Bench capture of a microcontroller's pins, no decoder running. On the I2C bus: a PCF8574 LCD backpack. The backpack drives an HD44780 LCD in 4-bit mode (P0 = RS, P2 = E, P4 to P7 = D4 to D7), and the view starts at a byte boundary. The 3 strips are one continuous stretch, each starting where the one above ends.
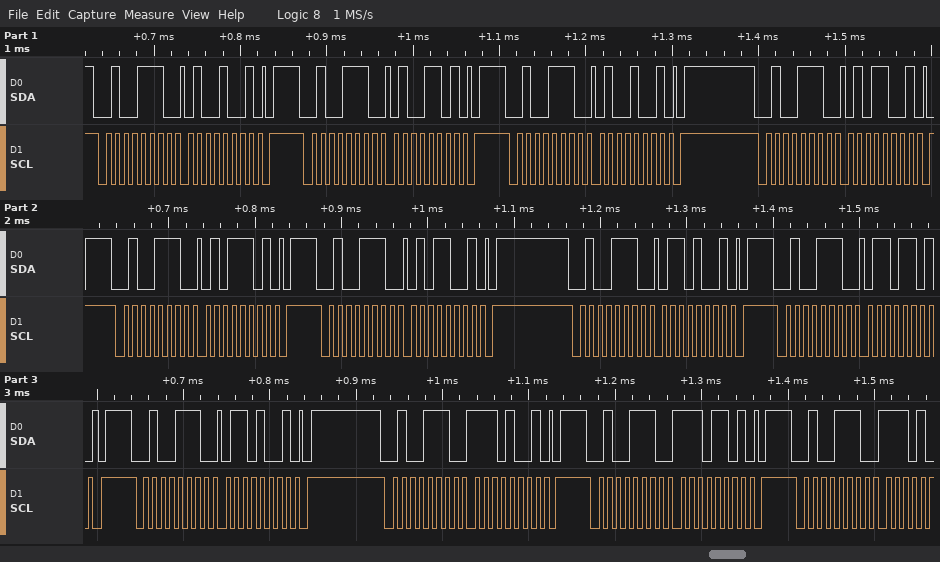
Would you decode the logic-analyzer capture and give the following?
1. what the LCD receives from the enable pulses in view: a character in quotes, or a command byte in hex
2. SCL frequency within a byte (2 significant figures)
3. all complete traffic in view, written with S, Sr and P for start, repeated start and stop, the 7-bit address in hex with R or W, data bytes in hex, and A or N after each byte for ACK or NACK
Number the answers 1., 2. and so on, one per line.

1. 'E'
2. 100 kHz
3. S 27W A 49 A P S 27W A 4D A P S 27W A 49 A P S 27W A 59 A P S 27W A 5D A P S 27W A 59 A P S 27W A 69 A P S 27W A 6D A P S 27W A 69 A P S 27W A E9 A P S 27W A ED A P S 27W A
